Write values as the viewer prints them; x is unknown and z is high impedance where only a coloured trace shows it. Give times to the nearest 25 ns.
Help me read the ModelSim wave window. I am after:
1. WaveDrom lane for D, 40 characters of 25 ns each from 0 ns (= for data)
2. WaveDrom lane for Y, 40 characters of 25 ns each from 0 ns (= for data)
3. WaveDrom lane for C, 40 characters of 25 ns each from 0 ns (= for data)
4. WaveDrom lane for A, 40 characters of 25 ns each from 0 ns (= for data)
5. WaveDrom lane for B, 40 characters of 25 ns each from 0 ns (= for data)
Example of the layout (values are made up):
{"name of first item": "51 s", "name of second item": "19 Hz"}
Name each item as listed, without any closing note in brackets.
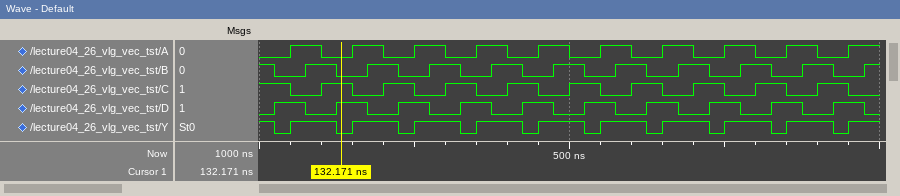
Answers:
{"WaveDrom lane for D, 40 characters of 25 ns each from 0 ns": "{name: 'D', wave: '01.0.1.0.1.0.1.0.1.0.1.0.1.0.1.0.1.0.1.0'}", "WaveDrom lane for Y, 40 characters of 25 ns each from 0 ns": "{name: 'Y', wave: '101..01..01..01..01..01..01..01..01..01.'}", "WaveDrom lane for C, 40 characters of 25 ns each from 0 ns": "{name: 'C', wave: '1.0.1.0.1.0.1.0.1.0.1.0.1.0.1.0.1.0.1.0.'}", "WaveDrom lane for A, 40 characters of 25 ns each from 0 ns": "{name: 'A', wave: '0.1.0.1.0.1.0.1.0.1.0.1.0.1.0.1.0.1.0.1.'}", "WaveDrom lane for B, 40 characters of 25 ns each from 0 ns": "{name: 'B', wave: '10.1.0.1.0.1.0.1.0.1.0.1.0.1.0.1.0.1.0.1'}"}
